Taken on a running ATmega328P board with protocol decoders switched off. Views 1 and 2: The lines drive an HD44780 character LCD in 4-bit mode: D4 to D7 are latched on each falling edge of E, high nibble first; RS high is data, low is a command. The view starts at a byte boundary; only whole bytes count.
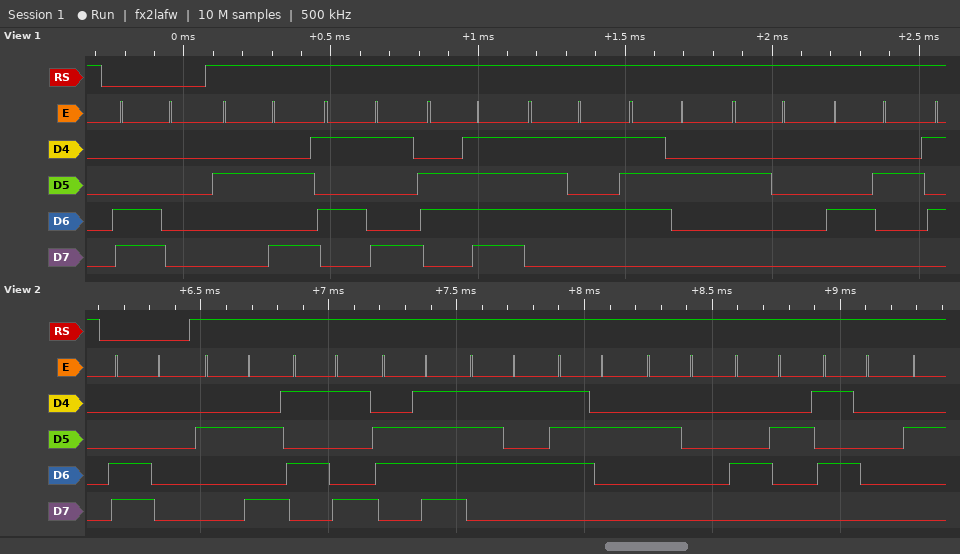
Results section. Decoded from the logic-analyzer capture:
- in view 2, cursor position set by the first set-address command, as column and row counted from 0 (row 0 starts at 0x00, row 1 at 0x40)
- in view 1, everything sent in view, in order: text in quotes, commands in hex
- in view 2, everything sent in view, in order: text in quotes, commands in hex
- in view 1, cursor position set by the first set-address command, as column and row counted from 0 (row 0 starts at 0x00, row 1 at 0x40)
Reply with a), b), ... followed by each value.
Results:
a) column 0, row 1
b) 0xC0 "*Your B"
c) 0xC0 "*Your BP"
d) column 0, row 1
